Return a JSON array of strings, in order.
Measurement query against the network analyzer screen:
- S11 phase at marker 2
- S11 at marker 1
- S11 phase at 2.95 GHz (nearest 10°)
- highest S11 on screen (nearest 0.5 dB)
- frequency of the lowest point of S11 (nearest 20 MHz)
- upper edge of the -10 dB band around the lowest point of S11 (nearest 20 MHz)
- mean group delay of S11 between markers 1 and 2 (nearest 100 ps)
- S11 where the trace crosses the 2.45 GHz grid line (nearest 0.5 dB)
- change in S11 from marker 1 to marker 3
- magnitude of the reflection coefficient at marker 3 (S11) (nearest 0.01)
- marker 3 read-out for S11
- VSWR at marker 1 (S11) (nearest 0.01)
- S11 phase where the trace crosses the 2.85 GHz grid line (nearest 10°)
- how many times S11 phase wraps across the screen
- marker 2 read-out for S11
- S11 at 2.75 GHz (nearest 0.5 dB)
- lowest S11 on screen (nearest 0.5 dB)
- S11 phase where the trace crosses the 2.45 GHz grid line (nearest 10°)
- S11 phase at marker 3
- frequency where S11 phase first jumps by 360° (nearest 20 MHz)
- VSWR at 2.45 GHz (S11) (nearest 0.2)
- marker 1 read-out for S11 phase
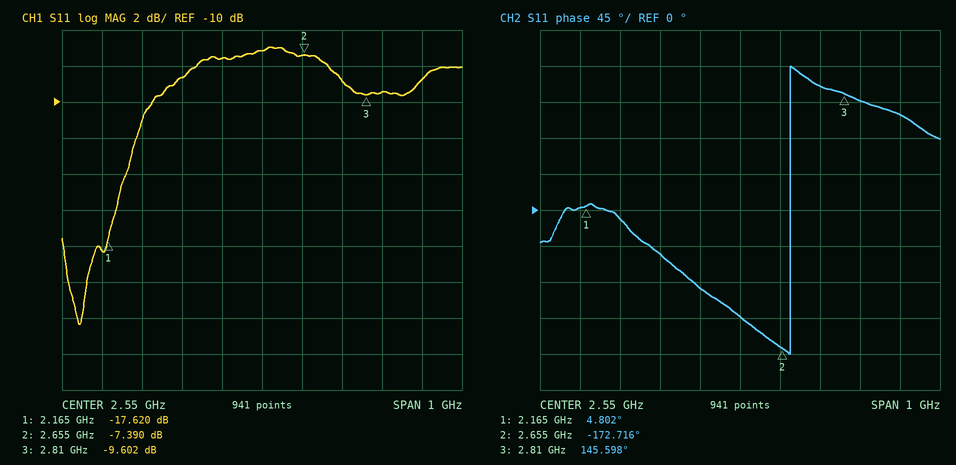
["-172.716°", "-17.620 dB", "120°", "-7.0 dB", "2.10 GHz", "2.28 GHz", "1.0 ns", "-7.5 dB", "8.018 dB", "0.33", "-9.602 dB", "1.30", "140°", "1", "-7.390 dB", "-9.0 dB", "-22.5 dB", "-100°", "145.598°", "2.68 GHz", "2.4", "4.802°"]
